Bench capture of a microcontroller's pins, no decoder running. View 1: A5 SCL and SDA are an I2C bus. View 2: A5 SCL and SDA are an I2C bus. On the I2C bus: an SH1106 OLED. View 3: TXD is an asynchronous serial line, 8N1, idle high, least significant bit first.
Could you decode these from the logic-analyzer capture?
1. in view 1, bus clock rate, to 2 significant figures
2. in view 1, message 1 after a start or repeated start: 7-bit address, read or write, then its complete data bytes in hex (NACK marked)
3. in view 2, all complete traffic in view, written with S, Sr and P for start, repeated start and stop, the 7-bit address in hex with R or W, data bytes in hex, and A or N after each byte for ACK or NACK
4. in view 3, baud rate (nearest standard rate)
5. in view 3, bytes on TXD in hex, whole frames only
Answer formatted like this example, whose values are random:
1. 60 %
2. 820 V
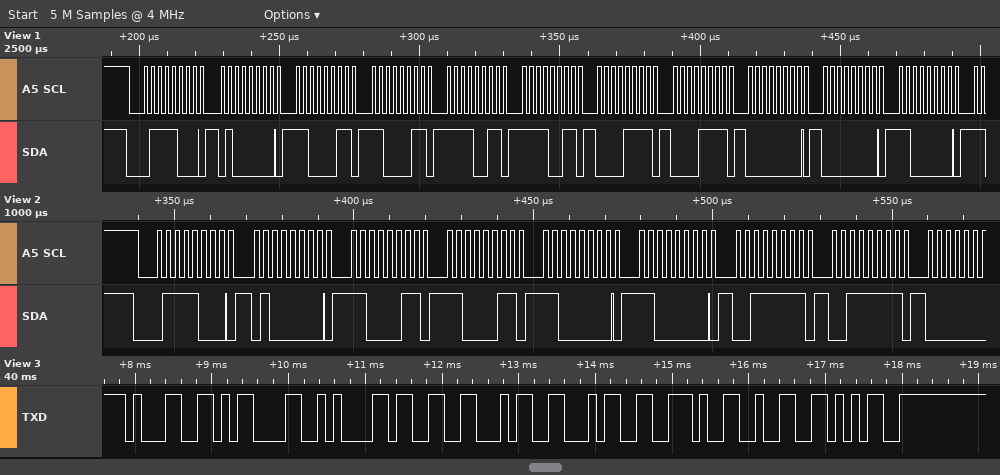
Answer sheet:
1. 400 kHz
2. 0x3C write: 40 C3 C3 F3 F3 0F 0F 00 00 C0
3. S 3CW A 40 A C3 A C3 A C0 A C0 A 3F A 3F A
4. 9600 baud
5. 31 0D 0A 33 34 34 2E 32 35
